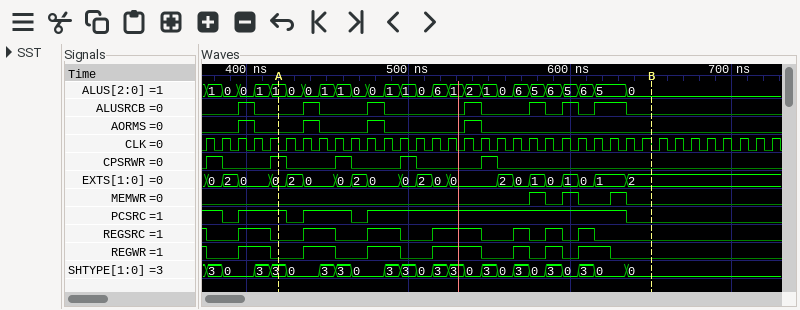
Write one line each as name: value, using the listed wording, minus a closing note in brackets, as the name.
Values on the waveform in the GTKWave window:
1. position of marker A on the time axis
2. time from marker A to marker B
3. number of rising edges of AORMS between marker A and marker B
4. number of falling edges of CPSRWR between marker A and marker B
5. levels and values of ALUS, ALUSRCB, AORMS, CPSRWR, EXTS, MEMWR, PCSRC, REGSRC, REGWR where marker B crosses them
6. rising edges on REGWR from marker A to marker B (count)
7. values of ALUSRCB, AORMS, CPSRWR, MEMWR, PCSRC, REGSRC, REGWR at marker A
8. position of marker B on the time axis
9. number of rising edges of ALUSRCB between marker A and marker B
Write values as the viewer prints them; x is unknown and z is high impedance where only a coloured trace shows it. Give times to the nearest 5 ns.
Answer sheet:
position of marker A on the time axis: 420 ns
time from marker A to marker B: 230 ns
number of rising edges of AORMS between marker A and marker B: 3
number of falling edges of CPSRWR between marker A and marker B: 4
levels and values of ALUS, ALUSRCB, AORMS, CPSRWR, EXTS, MEMWR, PCSRC, REGSRC, REGWR where marker B crosses them: ALUS=0, ALUSRCB=0, AORMS=0, CPSRWR=0, EXTS=2, MEMWR=0, PCSRC=0, REGSRC=0, REGWR=0
rising edges on REGWR from marker A to marker B: 6
values of ALUSRCB, AORMS, CPSRWR, MEMWR, PCSRC, REGSRC, REGWR at marker A: ALUSRCB=0, AORMS=0, CPSRWR=1, MEMWR=0, PCSRC=1, REGSRC=0, REGWR=0
position of marker B on the time axis: 650 ns
number of rising edges of ALUSRCB between marker A and marker B: 6
